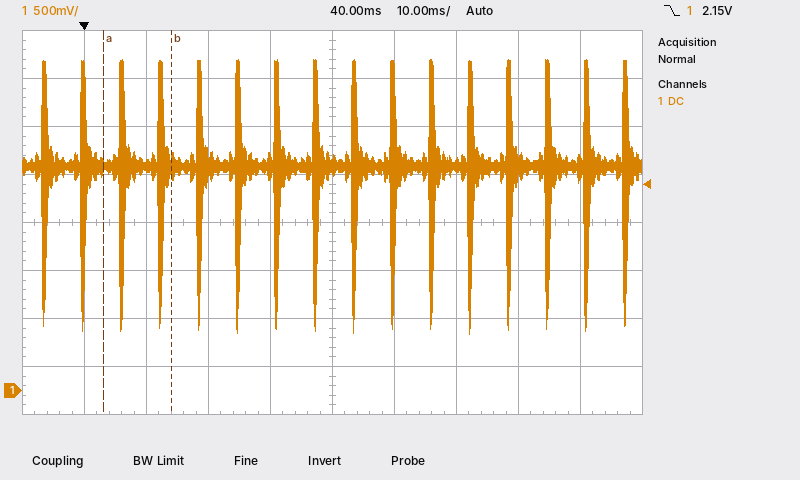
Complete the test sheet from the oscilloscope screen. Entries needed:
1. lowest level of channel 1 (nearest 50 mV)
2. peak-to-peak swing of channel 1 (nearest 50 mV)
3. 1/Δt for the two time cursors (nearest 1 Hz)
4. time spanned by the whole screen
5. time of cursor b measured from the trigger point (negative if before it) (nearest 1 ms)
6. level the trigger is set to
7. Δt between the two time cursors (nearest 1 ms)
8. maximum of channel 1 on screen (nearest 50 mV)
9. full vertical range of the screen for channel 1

600 mV
2.85 V
91 Hz
100 ms
+14 ms
2.15 V
11 ms
3.45 V
4 V
